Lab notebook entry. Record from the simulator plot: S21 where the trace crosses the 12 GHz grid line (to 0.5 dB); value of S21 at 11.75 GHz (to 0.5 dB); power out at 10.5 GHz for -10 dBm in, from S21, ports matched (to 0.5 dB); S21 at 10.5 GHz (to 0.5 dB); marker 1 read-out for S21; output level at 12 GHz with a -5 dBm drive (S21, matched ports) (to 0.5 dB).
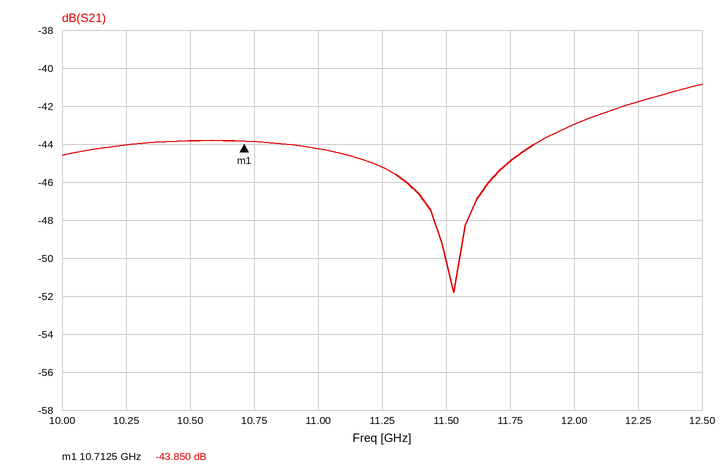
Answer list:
-43.0 dB
-45.0 dB
-54.0 dBm
-44.0 dB
-43.850 dB
-48.0 dBm
